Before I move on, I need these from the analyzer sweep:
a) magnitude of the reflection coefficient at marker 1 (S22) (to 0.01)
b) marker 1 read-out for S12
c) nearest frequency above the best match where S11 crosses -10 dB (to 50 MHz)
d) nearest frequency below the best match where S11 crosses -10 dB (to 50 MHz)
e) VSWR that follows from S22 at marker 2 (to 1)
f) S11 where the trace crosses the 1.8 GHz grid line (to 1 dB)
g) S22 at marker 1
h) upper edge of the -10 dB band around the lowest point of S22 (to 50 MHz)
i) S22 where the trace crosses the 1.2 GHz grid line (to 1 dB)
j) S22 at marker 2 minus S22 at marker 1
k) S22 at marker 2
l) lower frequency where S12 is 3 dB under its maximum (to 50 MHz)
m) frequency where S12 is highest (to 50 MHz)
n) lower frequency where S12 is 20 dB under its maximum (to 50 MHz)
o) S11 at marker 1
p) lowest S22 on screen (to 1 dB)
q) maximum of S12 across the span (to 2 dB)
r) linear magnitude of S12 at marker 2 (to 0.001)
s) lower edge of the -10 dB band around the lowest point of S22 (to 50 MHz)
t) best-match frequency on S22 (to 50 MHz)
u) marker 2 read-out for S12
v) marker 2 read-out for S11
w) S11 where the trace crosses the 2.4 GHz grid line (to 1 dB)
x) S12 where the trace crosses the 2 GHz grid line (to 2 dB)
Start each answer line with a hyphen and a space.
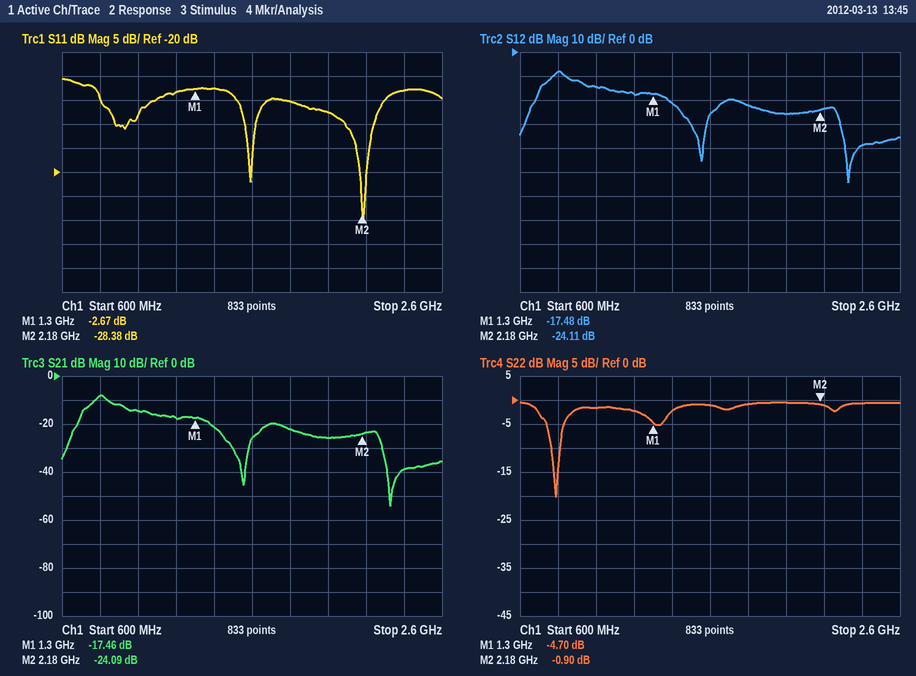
- 0.58
- -17.48 dB
- 2.25 GHz
- 2.10 GHz
- 19
- -5 dB
- -4.70 dB
- 800 MHz
- -2 dB
- 3.80 dB
- -0.90 dB
- 750 MHz
- 800 MHz
- 650 MHz
- -2.67 dB
- -20 dB
- -8 dB
- 0.062
- 750 MHz
- 800 MHz
- -24.11 dB
- -28.38 dB
- -3 dB
- -26 dB
